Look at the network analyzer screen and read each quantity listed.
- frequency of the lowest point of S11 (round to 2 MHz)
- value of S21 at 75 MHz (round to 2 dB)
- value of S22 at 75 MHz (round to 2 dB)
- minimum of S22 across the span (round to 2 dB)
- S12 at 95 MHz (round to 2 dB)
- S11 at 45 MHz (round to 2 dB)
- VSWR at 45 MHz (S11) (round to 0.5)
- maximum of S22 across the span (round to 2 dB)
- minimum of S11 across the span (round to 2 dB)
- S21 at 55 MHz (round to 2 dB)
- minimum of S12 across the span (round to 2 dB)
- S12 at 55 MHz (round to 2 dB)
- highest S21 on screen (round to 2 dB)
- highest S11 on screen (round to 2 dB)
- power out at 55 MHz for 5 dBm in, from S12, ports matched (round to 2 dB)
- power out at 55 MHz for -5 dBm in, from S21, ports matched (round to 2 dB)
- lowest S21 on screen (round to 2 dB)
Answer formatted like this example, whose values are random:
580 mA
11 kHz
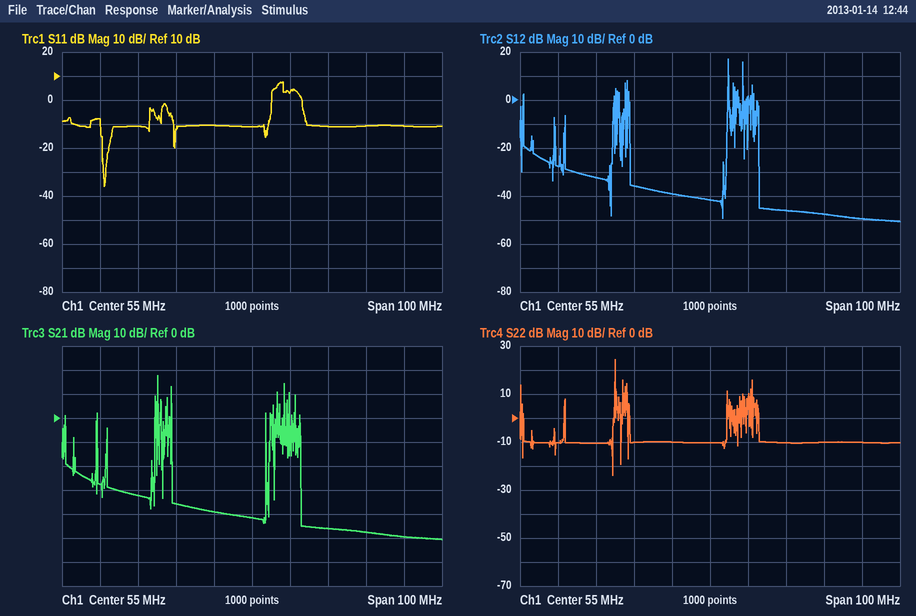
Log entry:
16 MHz
-46 dB
-10 dB
-24 dB
-50 dB
-10 dB
2.0
24 dB
-36 dB
-42 dB
-50 dB
-42 dB
18 dB
8 dB
-36 dBm
-46 dBm
-50 dB
